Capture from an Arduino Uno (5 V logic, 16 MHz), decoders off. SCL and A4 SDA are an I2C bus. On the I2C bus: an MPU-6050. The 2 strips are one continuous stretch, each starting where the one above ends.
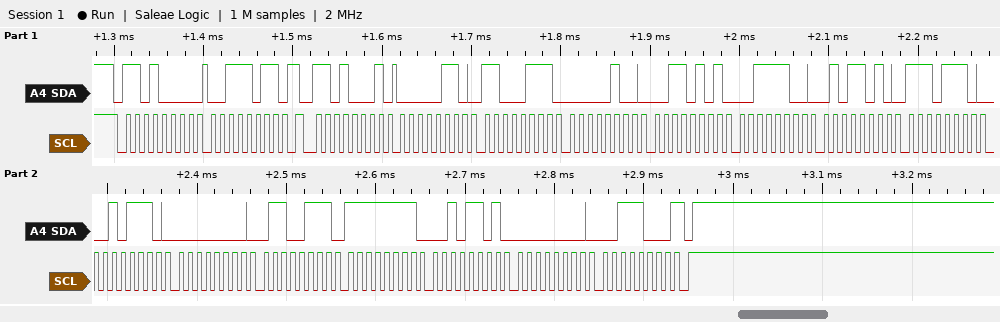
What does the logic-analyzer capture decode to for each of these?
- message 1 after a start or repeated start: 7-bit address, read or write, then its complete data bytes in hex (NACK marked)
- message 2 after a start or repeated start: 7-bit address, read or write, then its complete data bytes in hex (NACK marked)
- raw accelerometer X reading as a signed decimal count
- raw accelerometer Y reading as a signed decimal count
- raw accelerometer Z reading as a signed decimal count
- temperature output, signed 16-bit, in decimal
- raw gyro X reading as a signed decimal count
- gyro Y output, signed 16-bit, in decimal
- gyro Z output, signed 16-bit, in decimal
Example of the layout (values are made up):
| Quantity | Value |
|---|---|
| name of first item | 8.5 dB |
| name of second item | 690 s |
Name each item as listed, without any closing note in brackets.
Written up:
| Quantity | Value |
|---|---|
| message 1 after a start or repeated start: 7-bit address, read or write, then its complete data bytes in hex | 0x68 write: 3B |
| message 2 after a start or repeated start: 7-bit address, read or write, then its complete data bytes in hex | 0x68 read: 06 C7 04 35 3C 5A EE 2E 00 67 FF 2D 00 38 NACK |
| raw accelerometer X reading as a signed decimal count | 1735 |
| raw accelerometer Y reading as a signed decimal count | 1077 |
| raw accelerometer Z reading as a signed decimal count | 15450 |
| temperature output, signed 16-bit, in decimal | -4562 |
| raw gyro X reading as a signed decimal count | 103 |
| gyro Y output, signed 16-bit, in decimal | -211 |
| gyro Z output, signed 16-bit, in decimal | 56 |
